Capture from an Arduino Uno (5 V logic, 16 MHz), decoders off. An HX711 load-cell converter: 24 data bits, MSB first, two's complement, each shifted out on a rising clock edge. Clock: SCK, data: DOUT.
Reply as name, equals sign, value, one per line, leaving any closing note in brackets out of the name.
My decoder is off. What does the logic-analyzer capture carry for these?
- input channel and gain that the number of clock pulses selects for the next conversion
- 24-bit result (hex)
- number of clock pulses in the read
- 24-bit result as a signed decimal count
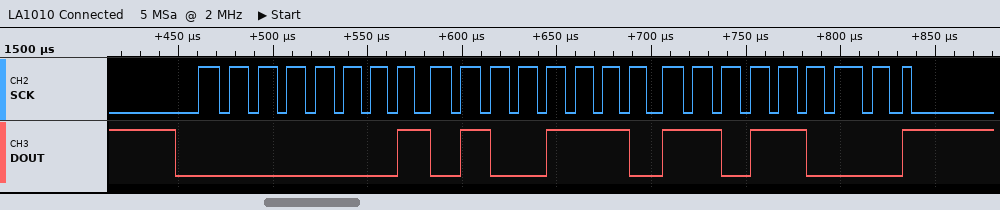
input channel and gain that the number of clock pulses selects for the next conversion = channel A, gain 128
24-bit result = 0x014ED8
number of clock pulses in the read = 25
24-bit result as a signed decimal count = 85720
